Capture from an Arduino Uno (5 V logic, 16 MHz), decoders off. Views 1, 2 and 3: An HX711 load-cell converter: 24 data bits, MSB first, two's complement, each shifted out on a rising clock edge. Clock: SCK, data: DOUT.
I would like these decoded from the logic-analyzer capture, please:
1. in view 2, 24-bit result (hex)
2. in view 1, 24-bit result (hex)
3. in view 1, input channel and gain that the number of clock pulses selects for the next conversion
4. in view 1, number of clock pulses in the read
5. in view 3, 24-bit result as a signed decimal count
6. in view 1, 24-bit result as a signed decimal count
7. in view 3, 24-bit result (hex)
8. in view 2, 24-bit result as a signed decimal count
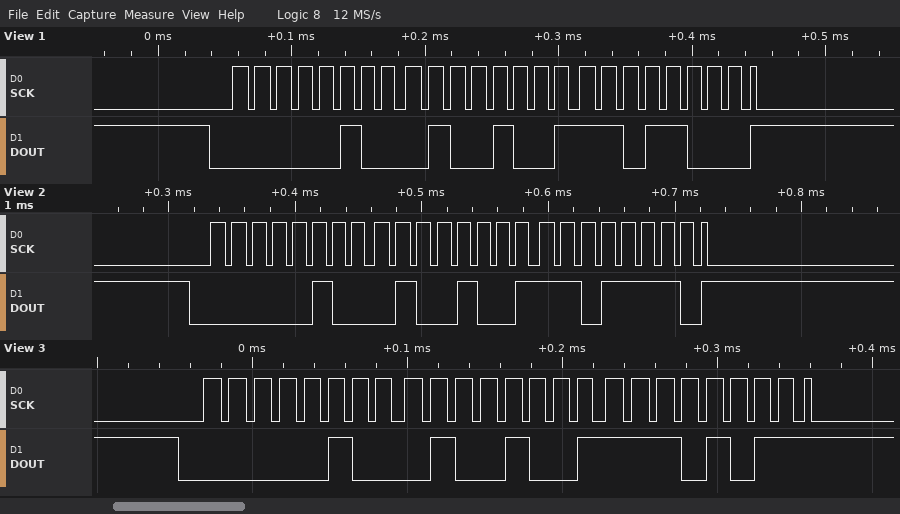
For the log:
0x0449DE
0x0449D8
channel A, gain 128
25
281067
281048
0x0449EB
281054
